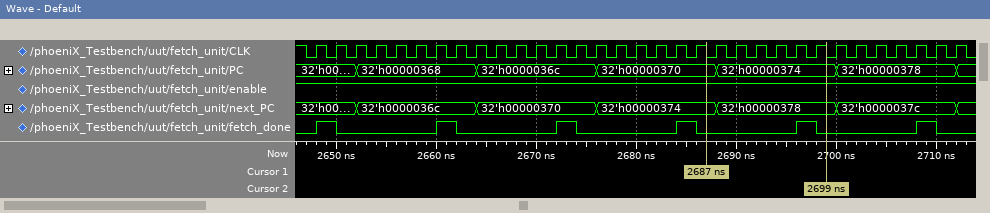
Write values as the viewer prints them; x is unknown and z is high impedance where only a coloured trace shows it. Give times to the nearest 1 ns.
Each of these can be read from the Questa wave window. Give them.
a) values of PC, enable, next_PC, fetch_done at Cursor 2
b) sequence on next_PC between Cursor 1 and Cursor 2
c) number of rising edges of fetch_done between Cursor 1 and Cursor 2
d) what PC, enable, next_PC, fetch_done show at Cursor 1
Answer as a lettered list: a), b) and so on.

a) PC=32'h00000374, enable=1, next_PC=32'h00000378, fetch_done=0
b) 32'h00000374, 32'h00000378
c) 1
d) PC=32'h00000370, enable=1, next_PC=32'h00000374, fetch_done=0
